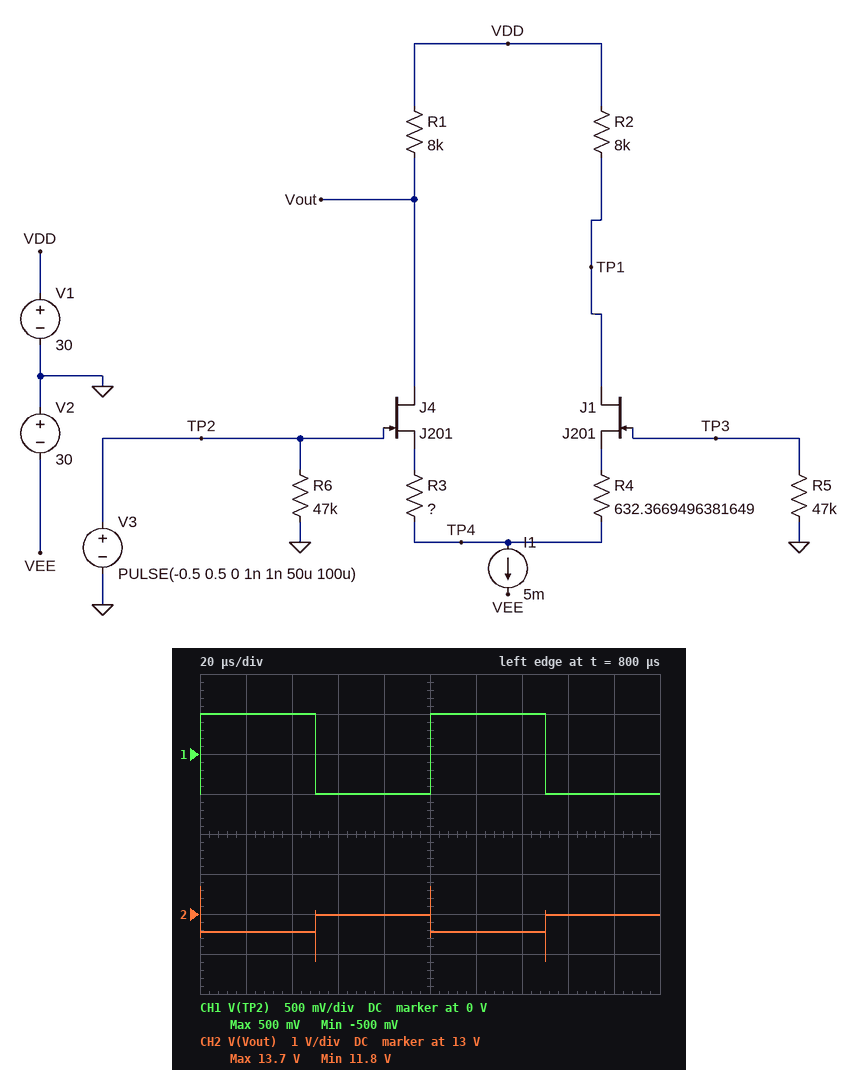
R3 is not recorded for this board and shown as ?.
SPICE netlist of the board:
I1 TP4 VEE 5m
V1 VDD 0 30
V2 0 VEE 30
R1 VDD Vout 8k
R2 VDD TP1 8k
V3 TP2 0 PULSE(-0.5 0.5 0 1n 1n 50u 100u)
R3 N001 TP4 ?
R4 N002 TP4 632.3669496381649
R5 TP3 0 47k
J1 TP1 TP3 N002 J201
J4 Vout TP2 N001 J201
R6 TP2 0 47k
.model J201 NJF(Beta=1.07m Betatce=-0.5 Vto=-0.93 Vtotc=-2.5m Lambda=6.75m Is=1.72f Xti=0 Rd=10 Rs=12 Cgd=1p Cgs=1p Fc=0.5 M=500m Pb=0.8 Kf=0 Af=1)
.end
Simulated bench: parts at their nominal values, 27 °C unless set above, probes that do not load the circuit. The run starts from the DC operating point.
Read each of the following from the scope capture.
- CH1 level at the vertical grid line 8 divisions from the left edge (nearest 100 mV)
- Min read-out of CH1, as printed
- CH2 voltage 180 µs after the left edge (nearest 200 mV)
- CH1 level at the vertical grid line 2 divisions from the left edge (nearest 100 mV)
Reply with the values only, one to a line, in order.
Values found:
-500 mV
-500 mV
13.0 V
500 mV
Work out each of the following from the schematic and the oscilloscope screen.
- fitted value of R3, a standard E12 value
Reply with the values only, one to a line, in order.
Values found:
2.2 kΩ
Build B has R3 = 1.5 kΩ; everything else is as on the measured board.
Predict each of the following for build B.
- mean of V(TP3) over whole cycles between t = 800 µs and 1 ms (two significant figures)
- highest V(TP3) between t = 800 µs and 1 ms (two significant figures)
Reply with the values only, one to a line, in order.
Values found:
-1.5 V
-1.1 V
